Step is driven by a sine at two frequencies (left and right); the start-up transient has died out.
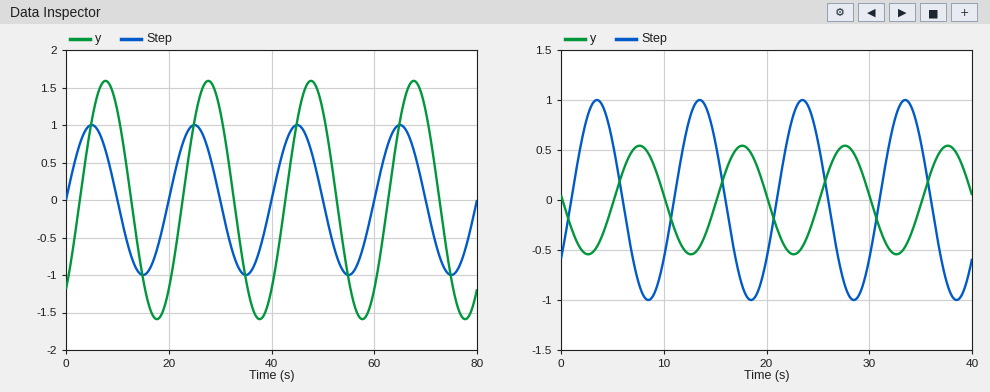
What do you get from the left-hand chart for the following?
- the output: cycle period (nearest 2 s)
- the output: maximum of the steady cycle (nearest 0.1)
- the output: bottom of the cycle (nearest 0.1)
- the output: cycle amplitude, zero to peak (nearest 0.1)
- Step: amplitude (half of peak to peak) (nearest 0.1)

20 s
1.6
-1.6
1.6
1.0
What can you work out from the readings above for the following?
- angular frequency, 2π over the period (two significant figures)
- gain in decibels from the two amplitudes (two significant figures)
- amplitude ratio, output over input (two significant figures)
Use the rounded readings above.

0.31 rad/s
4.1 dB
1.6
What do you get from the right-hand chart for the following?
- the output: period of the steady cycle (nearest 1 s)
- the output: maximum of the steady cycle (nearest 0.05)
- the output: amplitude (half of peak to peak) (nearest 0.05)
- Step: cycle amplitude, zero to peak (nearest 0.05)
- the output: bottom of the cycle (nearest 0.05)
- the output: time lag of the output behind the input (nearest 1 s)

10 s
0.55
0.55
1.00
-0.55
4 s
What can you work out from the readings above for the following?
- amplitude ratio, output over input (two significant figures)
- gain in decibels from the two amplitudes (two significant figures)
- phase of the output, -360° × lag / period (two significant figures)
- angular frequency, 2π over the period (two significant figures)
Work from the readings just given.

0.55
-5.2 dB
-140°
0.63 rad/s
